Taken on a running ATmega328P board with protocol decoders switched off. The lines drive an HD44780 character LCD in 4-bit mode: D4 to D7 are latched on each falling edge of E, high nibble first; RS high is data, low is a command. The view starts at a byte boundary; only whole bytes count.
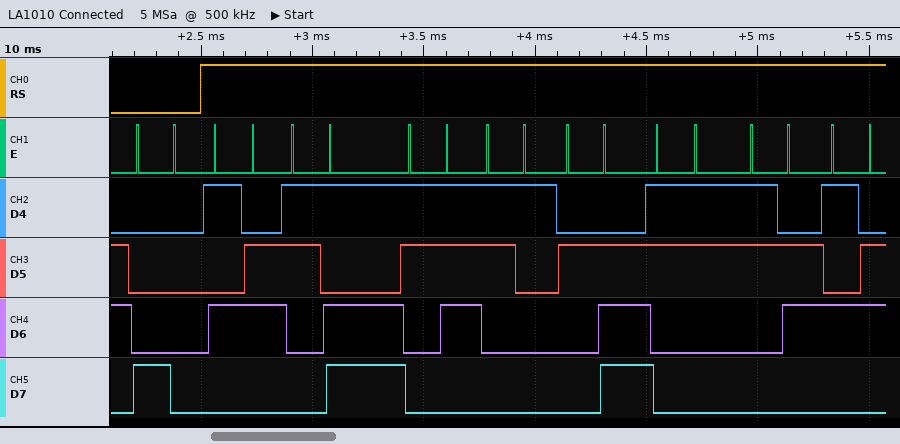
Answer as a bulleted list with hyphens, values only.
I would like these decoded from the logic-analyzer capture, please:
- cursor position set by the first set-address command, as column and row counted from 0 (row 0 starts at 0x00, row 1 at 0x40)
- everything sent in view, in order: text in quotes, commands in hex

- column 0, row 0
- 0x80 "V=71.36V"
